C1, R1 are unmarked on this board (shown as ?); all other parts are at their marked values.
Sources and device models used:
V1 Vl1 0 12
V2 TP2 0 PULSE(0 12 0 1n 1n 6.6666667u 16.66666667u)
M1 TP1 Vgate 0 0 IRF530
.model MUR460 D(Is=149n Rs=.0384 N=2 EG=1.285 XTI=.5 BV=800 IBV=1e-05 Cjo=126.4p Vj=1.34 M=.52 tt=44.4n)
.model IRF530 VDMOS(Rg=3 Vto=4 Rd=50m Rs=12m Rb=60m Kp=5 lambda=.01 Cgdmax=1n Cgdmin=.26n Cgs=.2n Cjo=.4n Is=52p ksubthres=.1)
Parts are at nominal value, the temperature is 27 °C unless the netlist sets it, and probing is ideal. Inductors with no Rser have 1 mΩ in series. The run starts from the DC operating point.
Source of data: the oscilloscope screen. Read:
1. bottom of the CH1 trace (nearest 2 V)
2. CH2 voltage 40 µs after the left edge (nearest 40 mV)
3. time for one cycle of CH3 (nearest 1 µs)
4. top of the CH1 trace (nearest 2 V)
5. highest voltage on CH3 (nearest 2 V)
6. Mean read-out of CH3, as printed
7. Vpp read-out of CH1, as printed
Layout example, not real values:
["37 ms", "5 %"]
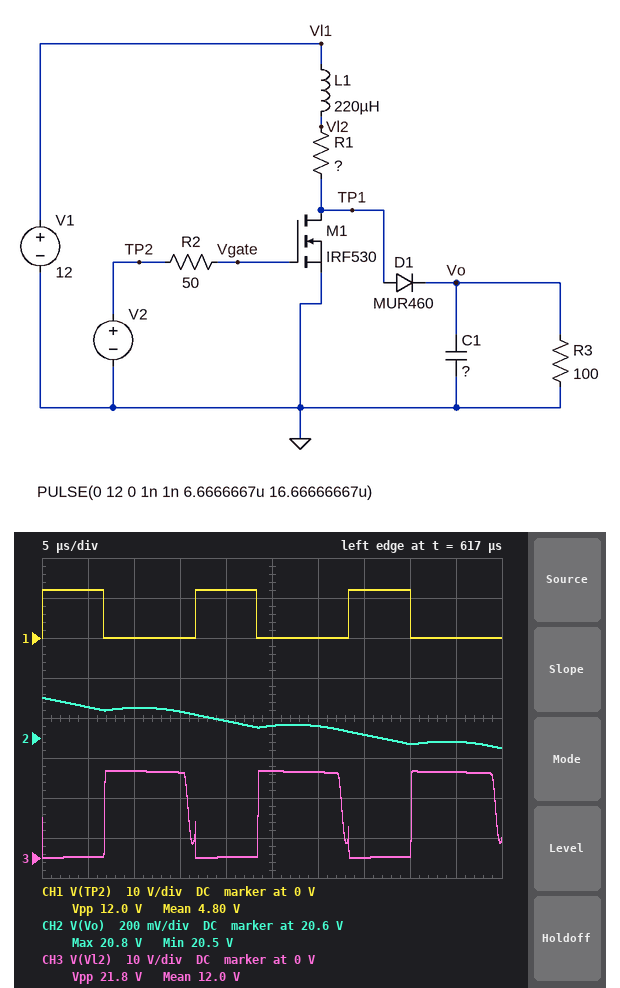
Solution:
["0 V", "20.56 V", "17 µs", "12 V", "22 V", "12.0 V", "12.0 V"]
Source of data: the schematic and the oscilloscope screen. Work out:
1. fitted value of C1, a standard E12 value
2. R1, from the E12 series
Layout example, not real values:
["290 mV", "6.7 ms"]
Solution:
["22 µF", "0.82 Ω"]
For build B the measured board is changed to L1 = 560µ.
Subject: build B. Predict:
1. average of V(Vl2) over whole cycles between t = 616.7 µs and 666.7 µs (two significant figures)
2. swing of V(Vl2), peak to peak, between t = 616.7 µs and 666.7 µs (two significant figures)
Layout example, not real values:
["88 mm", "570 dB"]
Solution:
["14 V", "24 V"]
